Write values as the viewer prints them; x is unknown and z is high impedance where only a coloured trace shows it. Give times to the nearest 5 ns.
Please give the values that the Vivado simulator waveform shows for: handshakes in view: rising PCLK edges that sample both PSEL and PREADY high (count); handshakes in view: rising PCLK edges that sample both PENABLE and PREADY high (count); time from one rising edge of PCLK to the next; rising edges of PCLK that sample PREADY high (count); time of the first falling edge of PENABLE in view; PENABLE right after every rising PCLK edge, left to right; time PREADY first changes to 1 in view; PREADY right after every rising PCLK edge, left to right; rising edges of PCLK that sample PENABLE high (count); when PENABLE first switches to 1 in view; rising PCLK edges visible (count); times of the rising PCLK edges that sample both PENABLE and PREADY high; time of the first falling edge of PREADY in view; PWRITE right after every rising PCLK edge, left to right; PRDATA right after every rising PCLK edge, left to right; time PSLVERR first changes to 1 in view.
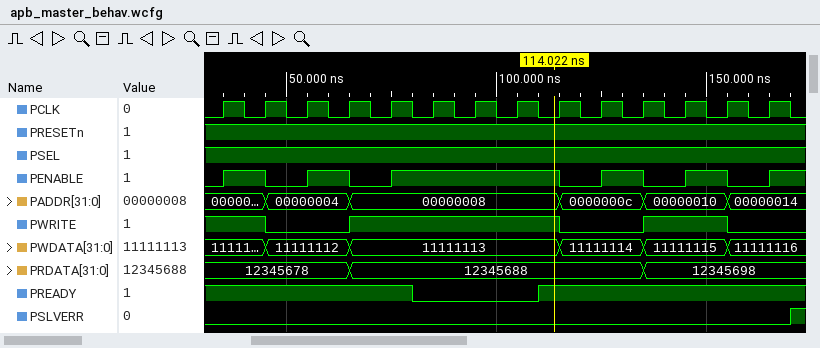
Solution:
11
5
10 ns
11
45 ns
1 0 1 0 1 1 1 1 0 1 0 1 0 1
110 ns
1 1 1 1 1 0 0 0 1 1 1 1 1 1
8
35 ns
14
45 ns, 65 ns, 115 ns, 135 ns, 155 ns
80 ns
1 0 0 1 1 1 1 1 0 0 1 1 0 0
12345678, 12345678, 12345678, 12345688, 12345688, 12345688, 12345688, 12345688, 12345688, 12345688, 12345698, 12345698, 12345698, 12345698
170 ns
